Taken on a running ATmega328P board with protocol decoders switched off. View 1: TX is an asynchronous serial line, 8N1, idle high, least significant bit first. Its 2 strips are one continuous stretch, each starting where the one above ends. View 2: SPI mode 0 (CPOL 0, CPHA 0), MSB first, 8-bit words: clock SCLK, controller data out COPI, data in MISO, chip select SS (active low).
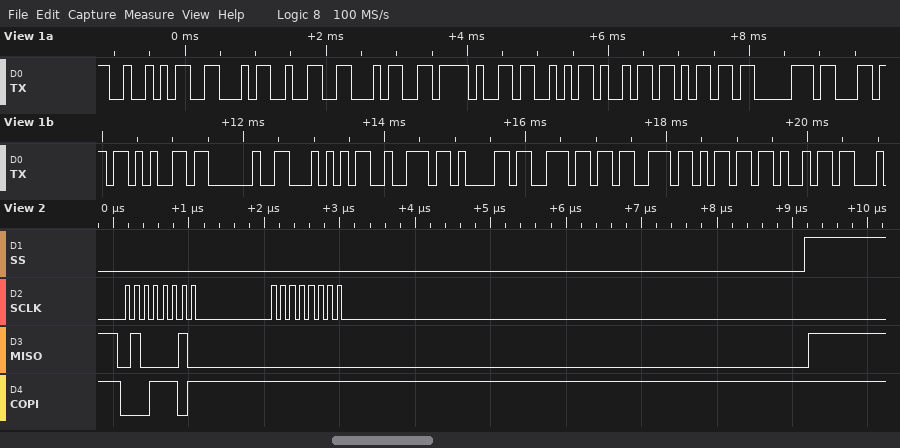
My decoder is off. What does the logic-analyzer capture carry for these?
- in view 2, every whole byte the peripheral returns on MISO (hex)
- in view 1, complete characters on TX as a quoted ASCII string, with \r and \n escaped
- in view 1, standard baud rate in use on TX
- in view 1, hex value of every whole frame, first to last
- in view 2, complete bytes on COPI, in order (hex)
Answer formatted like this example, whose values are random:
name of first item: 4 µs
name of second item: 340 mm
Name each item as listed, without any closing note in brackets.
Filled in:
in view 2, every whole byte the peripheral returns on MISO: 42 00
in view 1, complete characters on TX as a quoted ASCII string, with \r and \n escaped: "RF24/Simple Transmi"
in view 1, standard baud rate in use on TX: 9600 baud
in view 1, hex value of every whole frame, first to last: 0x52 0x46 0x32 0x34 0x2F 0x53 0x69 0x6D 0x70 0x6C 0x65 0x20 0x54 0x72 0x61 0x6E 0x73 0x6D 0x69
in view 2, complete bytes on COPI, in order: 1D FF
